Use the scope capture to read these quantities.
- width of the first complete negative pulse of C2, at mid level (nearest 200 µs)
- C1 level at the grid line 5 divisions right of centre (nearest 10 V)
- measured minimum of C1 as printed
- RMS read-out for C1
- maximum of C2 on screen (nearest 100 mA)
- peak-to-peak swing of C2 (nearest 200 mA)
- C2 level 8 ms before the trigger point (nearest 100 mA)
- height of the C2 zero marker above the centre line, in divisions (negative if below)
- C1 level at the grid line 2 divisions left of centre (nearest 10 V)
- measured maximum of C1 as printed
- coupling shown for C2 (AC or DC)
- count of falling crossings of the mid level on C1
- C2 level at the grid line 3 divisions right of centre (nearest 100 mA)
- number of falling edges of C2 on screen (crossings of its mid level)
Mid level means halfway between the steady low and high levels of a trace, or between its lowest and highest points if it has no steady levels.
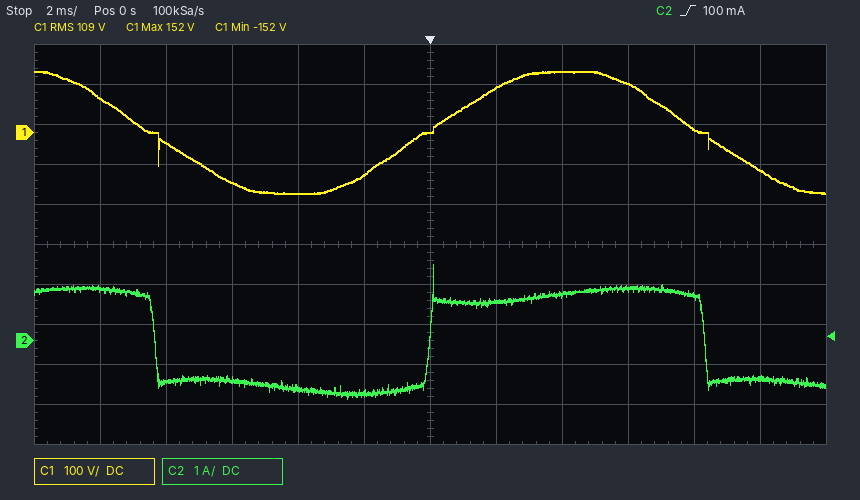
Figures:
8.4 ms
-90 V
-152 V
109 V
1.9 A
3.4 A
-1.0 A
-2.4 div
-150 V
152 V
DC
2
1.3 A
2
